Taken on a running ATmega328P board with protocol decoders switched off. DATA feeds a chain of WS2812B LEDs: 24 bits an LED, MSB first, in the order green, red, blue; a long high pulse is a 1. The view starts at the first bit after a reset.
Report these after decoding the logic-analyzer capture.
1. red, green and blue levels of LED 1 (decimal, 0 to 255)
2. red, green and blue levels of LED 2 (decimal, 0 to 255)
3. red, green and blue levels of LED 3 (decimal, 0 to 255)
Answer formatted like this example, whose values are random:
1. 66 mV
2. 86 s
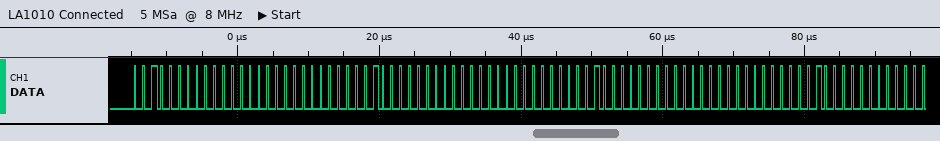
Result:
1. 0, 32, 0
2. 0, 16, 0
3. 0, 8, 0
